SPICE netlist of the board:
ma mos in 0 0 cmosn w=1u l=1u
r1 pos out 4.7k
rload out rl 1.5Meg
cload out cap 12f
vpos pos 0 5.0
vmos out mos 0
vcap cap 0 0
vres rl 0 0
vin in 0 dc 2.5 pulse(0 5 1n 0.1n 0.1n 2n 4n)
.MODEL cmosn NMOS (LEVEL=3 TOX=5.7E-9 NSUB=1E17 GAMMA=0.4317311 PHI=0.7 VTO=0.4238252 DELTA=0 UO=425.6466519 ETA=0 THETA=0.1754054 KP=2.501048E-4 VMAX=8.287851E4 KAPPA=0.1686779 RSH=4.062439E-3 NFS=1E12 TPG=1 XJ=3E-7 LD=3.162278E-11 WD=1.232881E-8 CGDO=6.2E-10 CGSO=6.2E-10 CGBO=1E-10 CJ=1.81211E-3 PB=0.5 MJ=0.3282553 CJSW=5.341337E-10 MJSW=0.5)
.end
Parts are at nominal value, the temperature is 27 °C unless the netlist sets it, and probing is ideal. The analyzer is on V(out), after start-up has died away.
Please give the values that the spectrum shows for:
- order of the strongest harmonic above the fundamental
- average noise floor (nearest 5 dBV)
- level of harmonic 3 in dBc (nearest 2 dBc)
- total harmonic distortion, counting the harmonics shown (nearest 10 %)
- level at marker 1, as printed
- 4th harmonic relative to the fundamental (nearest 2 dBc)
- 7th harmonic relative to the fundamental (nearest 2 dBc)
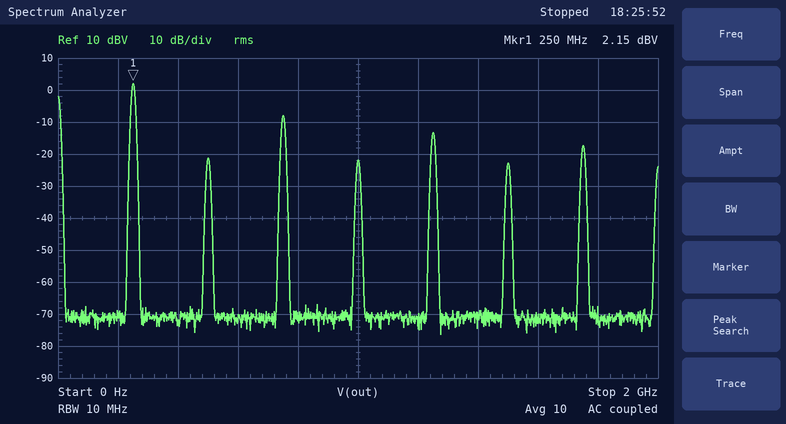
3
-70 dBV
-10 dBc
40 %
2.15 dBV
-24 dBc
-20 dBc
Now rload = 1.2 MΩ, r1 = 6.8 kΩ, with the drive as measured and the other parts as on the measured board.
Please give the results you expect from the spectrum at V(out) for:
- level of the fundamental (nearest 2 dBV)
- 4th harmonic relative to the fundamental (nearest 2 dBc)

4 dBV
-22 dBc
